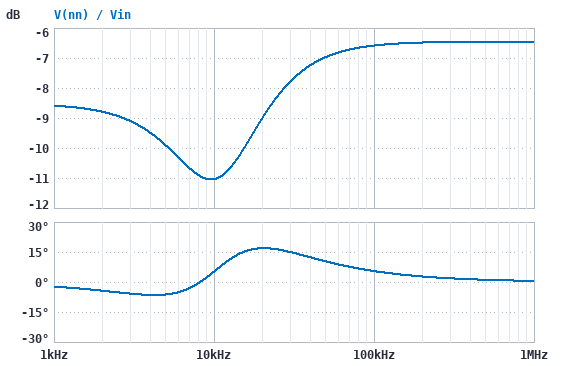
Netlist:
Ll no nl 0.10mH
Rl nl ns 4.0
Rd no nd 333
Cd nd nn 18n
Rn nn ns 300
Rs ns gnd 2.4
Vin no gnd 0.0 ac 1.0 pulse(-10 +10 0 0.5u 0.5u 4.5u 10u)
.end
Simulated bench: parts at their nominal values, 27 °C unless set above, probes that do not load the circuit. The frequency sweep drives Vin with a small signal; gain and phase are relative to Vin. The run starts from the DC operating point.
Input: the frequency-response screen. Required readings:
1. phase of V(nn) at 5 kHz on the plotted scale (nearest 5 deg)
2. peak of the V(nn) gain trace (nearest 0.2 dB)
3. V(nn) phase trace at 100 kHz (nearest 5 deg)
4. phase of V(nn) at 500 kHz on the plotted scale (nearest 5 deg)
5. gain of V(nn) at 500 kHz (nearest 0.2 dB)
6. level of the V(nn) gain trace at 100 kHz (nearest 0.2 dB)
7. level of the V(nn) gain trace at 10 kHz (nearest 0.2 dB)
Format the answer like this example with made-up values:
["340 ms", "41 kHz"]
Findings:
["-5 deg", "-6.4 dB", "5 deg", "0 deg", "-6.4 dB", "-6.6 dB", "-11.0 dB"]
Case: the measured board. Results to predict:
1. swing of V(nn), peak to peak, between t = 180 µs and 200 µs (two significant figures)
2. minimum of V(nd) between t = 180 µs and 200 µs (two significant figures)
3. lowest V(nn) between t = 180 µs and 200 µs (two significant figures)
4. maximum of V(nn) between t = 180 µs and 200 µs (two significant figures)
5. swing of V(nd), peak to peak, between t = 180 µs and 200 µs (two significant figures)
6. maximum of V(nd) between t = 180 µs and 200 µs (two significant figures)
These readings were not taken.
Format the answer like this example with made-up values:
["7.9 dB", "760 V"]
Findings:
["11 V", "-6.1 V", "-5.4 V", "5.4 V", "12 V", "6.1 V"]
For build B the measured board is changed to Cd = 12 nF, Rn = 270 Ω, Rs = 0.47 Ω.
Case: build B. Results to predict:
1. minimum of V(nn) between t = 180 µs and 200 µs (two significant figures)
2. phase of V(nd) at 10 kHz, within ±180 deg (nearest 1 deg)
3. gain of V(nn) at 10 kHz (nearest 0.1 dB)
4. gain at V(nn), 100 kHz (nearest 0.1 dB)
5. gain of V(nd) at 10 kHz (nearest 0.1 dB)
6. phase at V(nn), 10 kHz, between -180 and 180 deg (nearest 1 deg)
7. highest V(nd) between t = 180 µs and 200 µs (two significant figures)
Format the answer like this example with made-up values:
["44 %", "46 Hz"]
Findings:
["-5.7 V", "-13 deg", "-16.2 dB", "-7.2 dB", "-0.5 dB", "49 deg", "6.2 V"]
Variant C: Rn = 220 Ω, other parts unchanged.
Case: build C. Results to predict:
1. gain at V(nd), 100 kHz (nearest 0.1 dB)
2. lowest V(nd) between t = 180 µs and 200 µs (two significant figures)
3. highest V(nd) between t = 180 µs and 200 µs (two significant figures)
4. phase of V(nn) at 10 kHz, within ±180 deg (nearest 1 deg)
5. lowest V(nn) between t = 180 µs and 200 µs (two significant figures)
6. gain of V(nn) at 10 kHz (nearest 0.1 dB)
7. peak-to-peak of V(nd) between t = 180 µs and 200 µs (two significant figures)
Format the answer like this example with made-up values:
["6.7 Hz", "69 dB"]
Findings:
["-7.2 dB", "-5.7 V", "5.7 V", "-5 deg", "-4.5 V", "-12.1 dB", "11 V"]
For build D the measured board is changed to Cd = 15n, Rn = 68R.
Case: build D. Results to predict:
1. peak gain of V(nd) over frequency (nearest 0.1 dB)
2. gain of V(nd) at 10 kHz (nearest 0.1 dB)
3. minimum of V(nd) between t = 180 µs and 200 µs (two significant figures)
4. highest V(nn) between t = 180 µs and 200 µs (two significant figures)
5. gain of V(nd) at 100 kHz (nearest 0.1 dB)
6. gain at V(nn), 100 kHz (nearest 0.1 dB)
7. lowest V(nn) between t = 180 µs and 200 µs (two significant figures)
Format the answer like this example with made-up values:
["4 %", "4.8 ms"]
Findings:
["0.1 dB", "0 dB", "-5.2 V", "1.9 V", "-9.6 dB", "-15.6 dB", "-1.9 V"]
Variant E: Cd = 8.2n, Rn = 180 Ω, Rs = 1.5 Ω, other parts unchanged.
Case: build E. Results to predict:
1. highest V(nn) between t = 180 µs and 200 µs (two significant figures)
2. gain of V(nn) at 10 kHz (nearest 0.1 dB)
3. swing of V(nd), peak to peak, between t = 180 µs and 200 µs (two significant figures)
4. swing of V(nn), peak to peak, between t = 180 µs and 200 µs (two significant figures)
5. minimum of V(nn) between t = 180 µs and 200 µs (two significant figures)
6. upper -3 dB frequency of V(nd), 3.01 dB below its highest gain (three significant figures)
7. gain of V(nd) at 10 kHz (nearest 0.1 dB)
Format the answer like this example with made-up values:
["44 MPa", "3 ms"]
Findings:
["4.9 V", "-17.2 dB", "14 V", "9.7 V", "-4.9 V", "46.8 kHz", "0 dB"]
